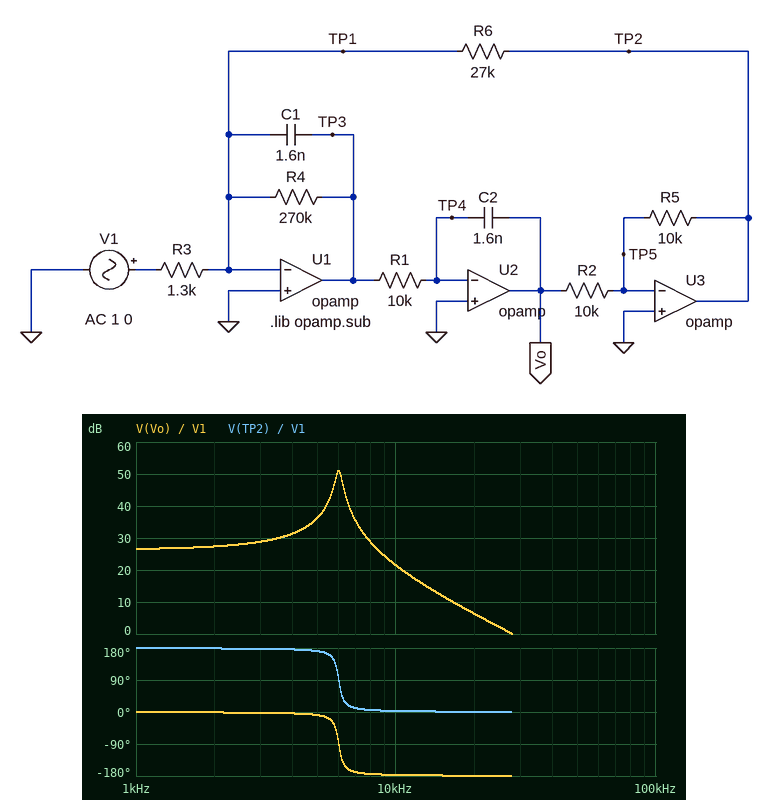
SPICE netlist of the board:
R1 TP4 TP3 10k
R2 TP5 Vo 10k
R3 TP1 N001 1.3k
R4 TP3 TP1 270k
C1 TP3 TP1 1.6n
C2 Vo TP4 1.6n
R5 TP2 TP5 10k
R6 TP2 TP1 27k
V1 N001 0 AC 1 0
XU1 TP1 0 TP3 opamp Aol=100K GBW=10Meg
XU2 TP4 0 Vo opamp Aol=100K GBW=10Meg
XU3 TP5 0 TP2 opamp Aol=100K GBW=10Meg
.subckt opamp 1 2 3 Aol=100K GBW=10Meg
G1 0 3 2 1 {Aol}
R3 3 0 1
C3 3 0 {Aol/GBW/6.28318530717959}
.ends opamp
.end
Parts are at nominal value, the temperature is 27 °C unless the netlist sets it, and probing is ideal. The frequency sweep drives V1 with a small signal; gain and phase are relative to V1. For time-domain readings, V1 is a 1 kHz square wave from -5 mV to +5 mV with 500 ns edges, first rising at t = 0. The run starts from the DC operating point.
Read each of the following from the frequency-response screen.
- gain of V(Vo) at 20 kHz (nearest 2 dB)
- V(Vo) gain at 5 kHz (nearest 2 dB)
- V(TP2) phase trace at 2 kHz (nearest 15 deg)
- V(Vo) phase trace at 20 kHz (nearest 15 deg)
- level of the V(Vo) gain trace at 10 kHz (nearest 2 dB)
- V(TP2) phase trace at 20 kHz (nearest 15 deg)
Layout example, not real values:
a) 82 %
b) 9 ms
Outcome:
a) 6 dB
b) 36 dB
c) 180 deg
d) -180 deg
e) 22 dB
f) 0 deg
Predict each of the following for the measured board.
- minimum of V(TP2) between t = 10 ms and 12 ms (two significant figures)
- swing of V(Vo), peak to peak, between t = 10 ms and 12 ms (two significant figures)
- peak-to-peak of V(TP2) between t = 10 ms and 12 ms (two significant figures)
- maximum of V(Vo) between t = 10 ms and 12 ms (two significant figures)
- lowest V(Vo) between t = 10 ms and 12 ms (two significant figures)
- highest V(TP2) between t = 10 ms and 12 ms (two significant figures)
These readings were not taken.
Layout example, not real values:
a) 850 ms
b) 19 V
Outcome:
a) -220 mV
b) 450 mV
c) 450 mV
d) 220 mV
e) -220 mV
f) 220 mV
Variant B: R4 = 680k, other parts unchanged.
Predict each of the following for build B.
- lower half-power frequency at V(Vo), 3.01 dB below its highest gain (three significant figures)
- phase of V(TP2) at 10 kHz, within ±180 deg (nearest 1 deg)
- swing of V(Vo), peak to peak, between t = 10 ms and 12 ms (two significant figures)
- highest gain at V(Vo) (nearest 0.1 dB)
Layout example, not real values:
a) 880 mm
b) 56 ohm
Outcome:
a) 5.96 kHz
b) 1 deg
c) 430 mV
d) 59.6 dB
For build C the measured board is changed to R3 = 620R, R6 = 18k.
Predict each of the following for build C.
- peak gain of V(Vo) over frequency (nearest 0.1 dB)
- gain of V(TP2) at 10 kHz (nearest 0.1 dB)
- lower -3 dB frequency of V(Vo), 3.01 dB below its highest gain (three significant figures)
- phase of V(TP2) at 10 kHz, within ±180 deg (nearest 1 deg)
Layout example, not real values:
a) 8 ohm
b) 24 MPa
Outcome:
a) 55.9 dB
b) 30.6 dB
c) 7.17 kHz
d) 4 deg
